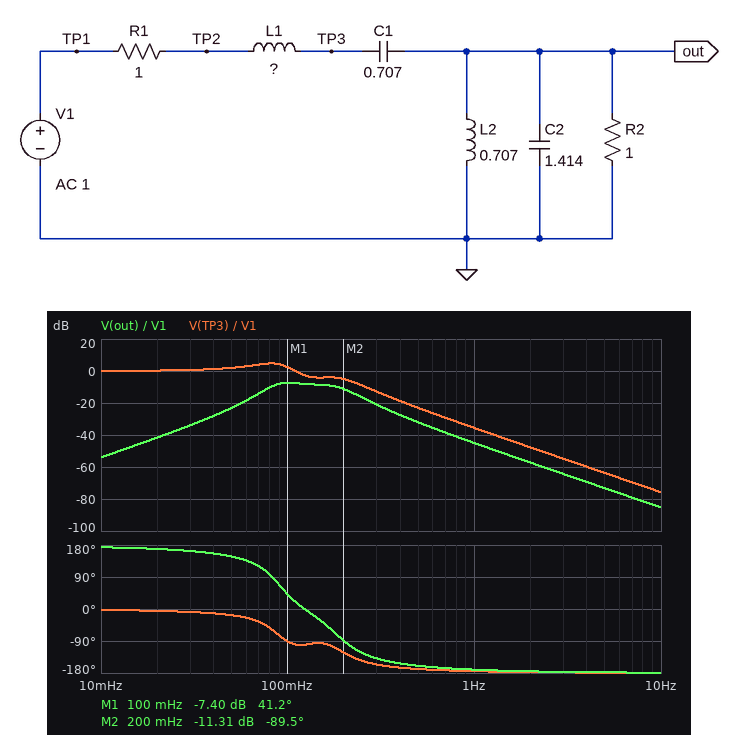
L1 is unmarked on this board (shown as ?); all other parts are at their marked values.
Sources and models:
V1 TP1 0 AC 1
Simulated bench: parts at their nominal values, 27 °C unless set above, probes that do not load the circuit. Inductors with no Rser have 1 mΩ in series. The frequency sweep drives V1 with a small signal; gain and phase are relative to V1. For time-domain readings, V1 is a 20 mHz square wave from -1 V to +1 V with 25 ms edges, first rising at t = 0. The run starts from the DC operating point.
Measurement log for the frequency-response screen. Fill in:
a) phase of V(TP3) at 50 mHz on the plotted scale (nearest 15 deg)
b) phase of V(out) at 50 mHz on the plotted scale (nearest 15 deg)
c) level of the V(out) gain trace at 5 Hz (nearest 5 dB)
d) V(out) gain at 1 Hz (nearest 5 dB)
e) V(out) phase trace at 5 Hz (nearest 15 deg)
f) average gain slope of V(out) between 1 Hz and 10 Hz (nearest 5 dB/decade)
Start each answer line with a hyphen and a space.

- -15 deg
- 150 deg
- -75 dB
- -45 dB
- -180 deg
- -40 dB/decade
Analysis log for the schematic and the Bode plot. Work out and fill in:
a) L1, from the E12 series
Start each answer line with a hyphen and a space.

- 3.3 H
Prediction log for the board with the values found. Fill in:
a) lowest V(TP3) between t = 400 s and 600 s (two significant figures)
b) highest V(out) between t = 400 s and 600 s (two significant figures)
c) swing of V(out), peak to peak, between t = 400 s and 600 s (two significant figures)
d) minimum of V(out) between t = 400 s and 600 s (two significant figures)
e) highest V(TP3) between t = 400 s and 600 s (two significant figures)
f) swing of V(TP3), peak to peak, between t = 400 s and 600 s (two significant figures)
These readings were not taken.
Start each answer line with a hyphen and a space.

- -1.5 V
- 260 mV
- 520 mV
- -260 mV
- 1.5 V
- 3.1 V
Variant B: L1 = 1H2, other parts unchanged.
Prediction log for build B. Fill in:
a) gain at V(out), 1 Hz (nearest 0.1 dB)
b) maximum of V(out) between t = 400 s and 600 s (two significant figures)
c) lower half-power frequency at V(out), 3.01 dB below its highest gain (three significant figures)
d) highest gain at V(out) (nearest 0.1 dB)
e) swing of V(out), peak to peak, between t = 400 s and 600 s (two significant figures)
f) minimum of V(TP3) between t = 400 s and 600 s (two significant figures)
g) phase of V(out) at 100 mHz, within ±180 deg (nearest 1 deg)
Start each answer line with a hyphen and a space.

- -36.0 dB
- 350 mV
- 100 mHz
- -6.1 dB
- 710 mV
- -1.2 V
- 91 deg
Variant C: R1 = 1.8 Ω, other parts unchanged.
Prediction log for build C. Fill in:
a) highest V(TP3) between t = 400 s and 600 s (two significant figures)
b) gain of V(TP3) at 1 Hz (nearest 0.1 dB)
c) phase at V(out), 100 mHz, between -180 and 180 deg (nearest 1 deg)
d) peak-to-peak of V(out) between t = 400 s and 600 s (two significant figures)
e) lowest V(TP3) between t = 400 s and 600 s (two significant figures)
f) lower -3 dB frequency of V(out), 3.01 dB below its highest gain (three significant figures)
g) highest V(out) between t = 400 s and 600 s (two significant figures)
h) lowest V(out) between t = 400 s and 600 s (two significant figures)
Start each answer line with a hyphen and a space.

- 1.3 V
- -35.6 dB
- 46 deg
- 420 mV
- -1.3 V
- 82.2 mHz
- 210 mV
- -210 mV
